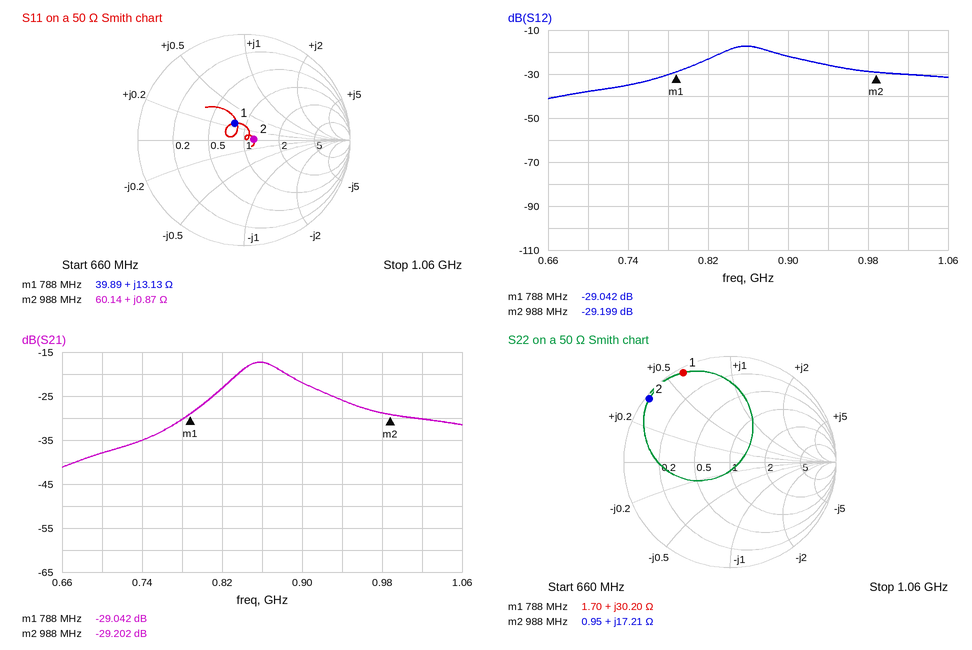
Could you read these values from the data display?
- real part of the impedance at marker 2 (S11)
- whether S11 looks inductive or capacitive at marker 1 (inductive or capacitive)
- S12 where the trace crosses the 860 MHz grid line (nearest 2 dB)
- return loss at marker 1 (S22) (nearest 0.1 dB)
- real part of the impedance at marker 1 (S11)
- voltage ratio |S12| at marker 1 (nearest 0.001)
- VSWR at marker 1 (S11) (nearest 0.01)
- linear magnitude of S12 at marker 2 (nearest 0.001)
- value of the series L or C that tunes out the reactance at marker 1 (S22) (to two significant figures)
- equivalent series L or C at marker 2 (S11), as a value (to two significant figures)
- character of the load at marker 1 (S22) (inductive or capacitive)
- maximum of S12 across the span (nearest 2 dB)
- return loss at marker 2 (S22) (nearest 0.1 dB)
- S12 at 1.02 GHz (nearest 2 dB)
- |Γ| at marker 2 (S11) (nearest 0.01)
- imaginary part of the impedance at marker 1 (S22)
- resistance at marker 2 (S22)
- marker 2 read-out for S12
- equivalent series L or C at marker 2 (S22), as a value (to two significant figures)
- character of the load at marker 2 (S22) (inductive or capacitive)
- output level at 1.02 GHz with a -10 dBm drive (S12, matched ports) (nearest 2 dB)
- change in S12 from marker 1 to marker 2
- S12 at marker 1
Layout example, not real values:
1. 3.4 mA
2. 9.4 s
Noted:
1. 60.14 Ω
2. inductive
3. -18 dB
4. 0.4 dB
5. 39.89 Ω
6. 0.035
7. 1.45
8. 0.035
9. 6.7 pF
10. 140 pH
11. inductive
12. -18 dB
13. 0.3 dB
14. -30 dB
15. 0.09
16. +30.20 Ω
17. 0.95 Ω
18. -29.199 dB
19. 2.8 nH
20. inductive
21. -40 dBm
22. -0.157 dB
23. -29.042 dB
